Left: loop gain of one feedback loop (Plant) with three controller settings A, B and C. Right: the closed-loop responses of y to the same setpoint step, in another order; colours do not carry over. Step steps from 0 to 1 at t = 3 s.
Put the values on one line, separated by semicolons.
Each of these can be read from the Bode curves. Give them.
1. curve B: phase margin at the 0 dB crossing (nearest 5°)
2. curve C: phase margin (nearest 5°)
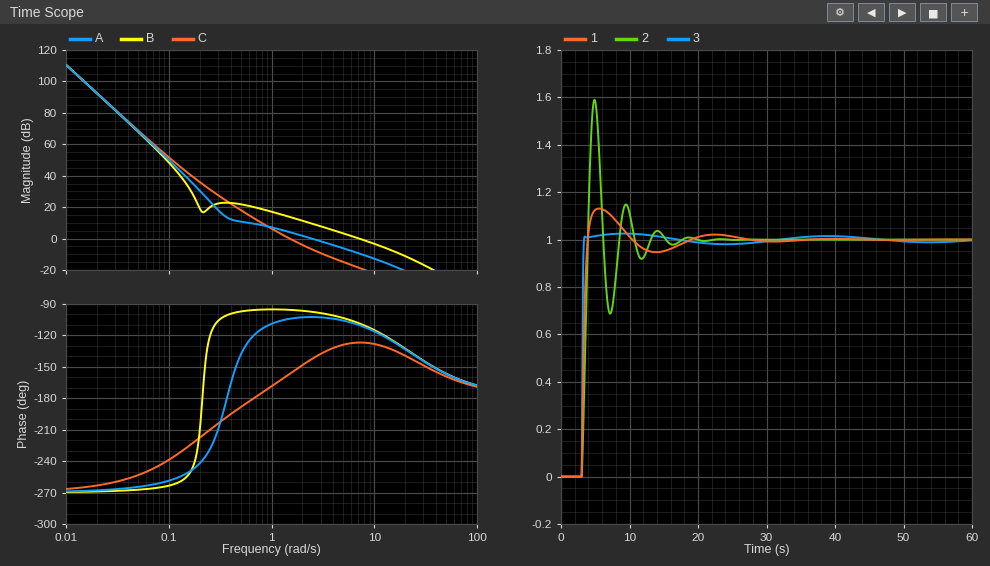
70°; 25°
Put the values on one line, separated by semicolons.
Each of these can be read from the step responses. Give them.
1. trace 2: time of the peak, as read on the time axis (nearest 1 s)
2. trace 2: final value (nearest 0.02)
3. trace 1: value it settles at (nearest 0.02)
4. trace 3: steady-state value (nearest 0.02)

5 s; 1.00; 1.00; 1.00
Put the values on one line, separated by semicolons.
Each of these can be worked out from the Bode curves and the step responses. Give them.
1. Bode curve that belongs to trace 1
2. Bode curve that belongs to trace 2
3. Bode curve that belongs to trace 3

A; C; B
